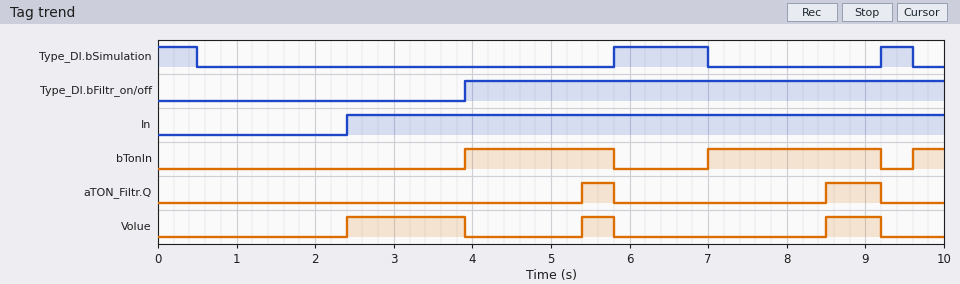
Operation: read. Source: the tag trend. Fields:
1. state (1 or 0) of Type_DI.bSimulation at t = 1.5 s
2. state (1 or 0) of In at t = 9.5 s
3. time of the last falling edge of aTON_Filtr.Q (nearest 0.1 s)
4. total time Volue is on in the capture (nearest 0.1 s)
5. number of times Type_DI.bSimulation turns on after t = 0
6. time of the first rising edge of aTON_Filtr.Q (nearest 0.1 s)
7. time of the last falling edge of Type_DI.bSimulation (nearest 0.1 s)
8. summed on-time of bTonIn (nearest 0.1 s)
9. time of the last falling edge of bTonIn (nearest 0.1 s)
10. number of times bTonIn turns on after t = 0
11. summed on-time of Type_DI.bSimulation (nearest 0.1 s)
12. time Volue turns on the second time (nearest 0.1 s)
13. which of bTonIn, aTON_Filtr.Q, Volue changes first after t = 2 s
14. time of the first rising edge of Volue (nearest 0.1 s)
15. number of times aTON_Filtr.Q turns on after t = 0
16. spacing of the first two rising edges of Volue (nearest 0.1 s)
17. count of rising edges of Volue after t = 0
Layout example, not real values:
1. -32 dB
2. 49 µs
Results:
1. 0
2. 1
3. 9.2 s
4. 2.6 s
5. 2
6. 5.4 s
7. 9.6 s
8. 4.5 s
9. 9.2 s
10. 3
11. 2.1 s
12. 5.4 s
13. Volue
14. 2.4 s
15. 2
16. 3.0 s
17. 3
